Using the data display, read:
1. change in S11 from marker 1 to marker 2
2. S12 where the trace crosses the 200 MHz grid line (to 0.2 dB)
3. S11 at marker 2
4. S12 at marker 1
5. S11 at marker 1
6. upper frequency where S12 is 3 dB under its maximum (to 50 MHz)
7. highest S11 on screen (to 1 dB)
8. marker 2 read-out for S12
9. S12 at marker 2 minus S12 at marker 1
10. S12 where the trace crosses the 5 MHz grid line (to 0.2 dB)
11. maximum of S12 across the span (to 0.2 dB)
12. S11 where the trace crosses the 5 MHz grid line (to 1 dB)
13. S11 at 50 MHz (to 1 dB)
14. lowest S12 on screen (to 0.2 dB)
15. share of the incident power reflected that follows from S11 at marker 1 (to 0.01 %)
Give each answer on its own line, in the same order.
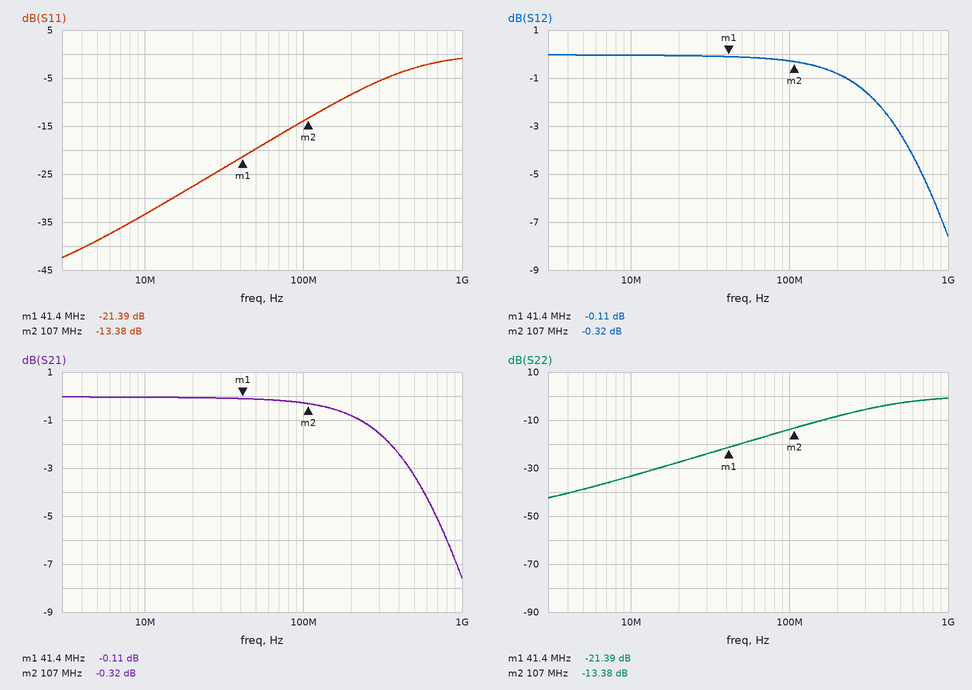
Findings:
8.01 dB
-0.8 dB
-13.38 dB
-0.11 dB
-21.39 dB
450 MHz
-1 dB
-0.32 dB
-0.21 dB
0.0 dB
0.0 dB
-39 dB
-20 dB
-7.6 dB
0.73 %
